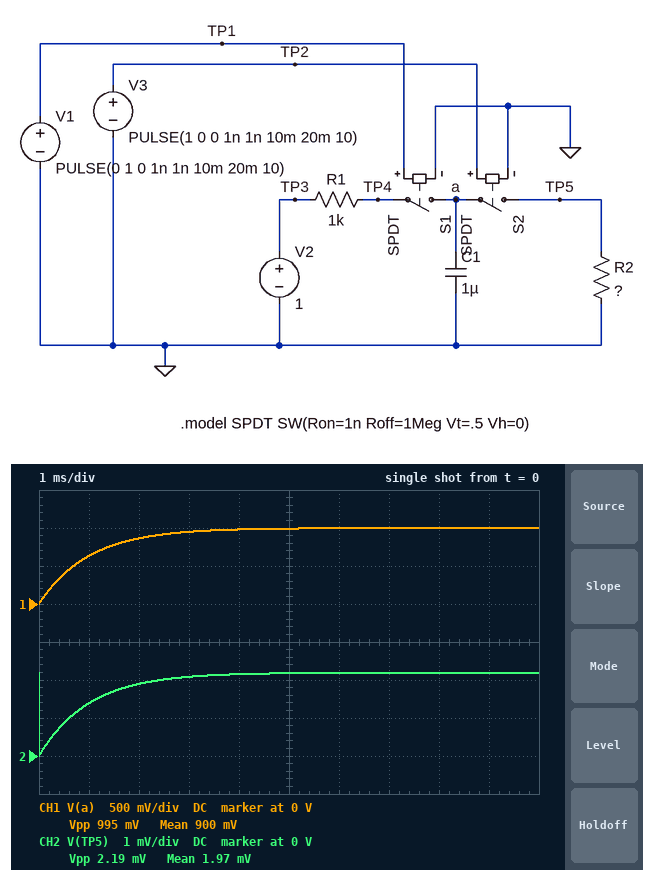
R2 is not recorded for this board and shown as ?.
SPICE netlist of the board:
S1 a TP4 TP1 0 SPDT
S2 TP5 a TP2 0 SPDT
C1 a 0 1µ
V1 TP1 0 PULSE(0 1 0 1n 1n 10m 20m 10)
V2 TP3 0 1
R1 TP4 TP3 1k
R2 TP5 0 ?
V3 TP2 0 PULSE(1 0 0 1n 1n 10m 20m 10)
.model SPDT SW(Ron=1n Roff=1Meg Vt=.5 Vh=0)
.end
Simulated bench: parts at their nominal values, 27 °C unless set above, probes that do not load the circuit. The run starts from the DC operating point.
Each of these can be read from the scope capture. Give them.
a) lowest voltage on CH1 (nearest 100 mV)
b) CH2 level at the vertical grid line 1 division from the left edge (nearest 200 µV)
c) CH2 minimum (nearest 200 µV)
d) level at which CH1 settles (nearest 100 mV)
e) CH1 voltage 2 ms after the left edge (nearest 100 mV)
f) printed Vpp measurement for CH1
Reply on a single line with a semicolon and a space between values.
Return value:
0 V; 1.4 mV; 0 V; 1.0 V; 900 mV; 995 mV
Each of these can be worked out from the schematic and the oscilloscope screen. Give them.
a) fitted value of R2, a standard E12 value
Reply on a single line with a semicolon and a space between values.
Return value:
2.2 kΩ
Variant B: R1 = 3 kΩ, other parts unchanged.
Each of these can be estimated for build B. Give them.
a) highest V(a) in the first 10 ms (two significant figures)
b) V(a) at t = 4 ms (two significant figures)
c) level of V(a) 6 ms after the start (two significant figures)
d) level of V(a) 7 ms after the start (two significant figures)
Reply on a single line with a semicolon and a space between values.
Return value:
960 mV; 740 mV; 860 mV; 900 mV
